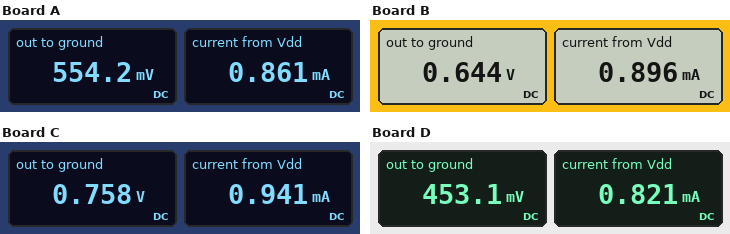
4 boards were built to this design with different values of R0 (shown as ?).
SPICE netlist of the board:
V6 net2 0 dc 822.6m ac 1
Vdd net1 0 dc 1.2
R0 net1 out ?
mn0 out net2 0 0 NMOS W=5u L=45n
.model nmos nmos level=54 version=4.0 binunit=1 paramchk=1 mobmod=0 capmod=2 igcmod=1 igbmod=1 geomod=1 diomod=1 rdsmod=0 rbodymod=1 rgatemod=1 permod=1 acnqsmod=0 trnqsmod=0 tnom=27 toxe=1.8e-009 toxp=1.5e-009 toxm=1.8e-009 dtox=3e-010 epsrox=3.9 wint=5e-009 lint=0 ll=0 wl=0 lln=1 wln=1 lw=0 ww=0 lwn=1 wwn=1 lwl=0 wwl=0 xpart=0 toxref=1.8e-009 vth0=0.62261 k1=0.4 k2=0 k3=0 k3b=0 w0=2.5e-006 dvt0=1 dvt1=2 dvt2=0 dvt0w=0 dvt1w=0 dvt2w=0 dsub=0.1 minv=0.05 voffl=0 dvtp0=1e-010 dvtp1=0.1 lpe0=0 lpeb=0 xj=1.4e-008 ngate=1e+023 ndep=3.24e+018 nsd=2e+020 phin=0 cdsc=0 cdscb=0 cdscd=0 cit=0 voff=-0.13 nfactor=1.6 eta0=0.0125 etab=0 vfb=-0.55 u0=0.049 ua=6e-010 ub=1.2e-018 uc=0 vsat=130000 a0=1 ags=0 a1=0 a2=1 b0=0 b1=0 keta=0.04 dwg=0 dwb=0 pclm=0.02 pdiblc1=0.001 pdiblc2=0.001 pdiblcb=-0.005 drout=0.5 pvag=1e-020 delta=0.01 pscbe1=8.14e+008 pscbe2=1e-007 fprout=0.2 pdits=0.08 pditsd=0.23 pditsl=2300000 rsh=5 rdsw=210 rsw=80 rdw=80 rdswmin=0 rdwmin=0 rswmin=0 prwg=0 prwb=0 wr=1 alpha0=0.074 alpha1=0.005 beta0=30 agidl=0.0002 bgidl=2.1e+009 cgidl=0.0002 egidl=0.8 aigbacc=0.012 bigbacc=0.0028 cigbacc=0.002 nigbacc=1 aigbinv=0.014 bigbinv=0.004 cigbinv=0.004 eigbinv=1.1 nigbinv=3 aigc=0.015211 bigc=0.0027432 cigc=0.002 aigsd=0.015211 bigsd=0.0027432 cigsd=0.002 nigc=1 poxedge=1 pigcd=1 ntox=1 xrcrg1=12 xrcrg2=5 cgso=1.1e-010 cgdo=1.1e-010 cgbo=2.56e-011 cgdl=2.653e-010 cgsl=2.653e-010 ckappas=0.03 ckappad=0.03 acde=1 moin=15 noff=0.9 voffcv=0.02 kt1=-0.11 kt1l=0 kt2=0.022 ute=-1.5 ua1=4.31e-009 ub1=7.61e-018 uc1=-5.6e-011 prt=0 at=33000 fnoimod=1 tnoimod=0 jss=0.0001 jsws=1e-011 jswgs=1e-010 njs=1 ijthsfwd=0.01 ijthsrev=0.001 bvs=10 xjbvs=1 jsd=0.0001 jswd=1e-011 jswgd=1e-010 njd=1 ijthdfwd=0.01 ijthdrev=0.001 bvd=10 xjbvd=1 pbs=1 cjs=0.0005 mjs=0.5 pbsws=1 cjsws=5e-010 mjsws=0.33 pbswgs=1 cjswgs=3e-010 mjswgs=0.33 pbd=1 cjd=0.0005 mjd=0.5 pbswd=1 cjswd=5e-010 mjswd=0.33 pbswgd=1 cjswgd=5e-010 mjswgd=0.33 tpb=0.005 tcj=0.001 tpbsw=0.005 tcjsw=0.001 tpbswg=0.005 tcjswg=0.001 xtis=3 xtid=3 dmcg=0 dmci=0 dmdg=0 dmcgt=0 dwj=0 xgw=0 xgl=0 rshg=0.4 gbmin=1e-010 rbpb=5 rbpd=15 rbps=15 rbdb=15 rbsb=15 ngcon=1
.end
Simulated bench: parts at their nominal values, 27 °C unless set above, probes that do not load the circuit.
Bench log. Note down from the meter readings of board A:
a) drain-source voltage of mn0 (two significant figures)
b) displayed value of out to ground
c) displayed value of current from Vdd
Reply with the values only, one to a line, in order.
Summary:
550 mV
554.2 mV
0.861 mA
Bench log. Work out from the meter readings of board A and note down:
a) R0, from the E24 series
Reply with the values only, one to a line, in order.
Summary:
750 Ω
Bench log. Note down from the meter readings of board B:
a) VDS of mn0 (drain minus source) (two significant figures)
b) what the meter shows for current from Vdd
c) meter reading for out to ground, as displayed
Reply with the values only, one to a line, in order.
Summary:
640 mV
0.896 mA
0.644 V
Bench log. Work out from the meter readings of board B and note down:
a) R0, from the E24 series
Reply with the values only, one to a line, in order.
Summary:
620 Ω
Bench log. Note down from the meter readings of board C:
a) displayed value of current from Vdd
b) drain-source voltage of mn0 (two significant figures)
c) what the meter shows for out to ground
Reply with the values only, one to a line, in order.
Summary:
0.941 mA
760 mV
0.758 V
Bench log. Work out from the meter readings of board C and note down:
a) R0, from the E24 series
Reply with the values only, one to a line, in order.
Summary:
470 Ω
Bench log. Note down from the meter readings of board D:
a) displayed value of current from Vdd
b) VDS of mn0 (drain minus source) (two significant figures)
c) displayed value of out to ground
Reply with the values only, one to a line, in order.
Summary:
0.821 mA
450 mV
453.1 mV
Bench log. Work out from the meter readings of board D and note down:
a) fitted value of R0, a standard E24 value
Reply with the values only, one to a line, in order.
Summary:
910 Ω
